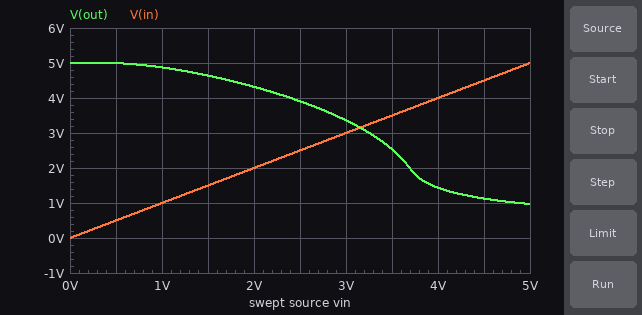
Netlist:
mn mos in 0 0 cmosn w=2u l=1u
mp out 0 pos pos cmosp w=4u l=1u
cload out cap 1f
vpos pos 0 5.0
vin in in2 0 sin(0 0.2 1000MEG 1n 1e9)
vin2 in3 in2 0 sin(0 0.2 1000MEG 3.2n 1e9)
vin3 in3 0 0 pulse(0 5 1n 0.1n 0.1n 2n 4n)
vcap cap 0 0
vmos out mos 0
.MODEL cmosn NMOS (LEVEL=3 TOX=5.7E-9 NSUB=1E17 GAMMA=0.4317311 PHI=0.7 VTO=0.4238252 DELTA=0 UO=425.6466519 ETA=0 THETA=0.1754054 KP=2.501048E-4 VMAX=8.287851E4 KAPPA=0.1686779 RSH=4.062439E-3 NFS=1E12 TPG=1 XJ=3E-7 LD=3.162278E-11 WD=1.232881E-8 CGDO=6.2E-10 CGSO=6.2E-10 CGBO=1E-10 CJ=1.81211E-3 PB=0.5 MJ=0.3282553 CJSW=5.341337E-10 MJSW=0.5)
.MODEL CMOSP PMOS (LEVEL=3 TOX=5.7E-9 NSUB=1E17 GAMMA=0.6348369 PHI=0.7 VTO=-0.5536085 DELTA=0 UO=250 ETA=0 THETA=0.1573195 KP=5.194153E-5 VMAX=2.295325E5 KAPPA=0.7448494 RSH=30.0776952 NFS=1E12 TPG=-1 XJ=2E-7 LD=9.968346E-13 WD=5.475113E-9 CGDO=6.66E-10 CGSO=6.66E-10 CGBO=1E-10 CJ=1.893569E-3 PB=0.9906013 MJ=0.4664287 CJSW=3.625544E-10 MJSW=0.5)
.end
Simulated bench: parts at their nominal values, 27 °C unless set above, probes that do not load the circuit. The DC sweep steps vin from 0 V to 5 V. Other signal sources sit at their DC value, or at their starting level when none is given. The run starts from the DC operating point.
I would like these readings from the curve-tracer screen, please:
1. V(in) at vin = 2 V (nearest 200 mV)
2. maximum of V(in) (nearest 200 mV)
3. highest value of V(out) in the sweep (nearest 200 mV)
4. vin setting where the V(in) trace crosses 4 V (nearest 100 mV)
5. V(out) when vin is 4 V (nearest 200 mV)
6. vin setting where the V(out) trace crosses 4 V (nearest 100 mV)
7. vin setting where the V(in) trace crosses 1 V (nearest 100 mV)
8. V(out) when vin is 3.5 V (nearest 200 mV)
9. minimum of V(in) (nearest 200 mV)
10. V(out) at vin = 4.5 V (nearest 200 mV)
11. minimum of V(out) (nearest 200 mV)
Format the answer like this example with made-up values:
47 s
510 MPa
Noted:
2.0 V
5.0 V
5.0 V
4.0 V
1.4 V
2.4 V
1.0 V
2.6 V
0 V
1.2 V
1.0 V
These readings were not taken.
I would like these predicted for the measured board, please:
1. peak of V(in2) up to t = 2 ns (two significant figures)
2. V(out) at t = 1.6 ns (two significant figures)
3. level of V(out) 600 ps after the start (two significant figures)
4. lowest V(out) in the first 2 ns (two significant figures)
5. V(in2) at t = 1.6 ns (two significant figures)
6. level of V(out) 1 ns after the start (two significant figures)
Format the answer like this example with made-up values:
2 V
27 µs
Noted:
5.0 V
980 mV
5.0 V
930 mV
5.0 V
5.0 V
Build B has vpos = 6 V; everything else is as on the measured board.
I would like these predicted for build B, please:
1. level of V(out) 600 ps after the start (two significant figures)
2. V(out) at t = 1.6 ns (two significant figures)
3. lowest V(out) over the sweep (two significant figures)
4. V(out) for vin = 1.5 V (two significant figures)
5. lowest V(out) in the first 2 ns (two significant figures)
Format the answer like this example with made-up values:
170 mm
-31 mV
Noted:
6.0 V
1.7 V
1.6 V
5.7 V
1.5 V
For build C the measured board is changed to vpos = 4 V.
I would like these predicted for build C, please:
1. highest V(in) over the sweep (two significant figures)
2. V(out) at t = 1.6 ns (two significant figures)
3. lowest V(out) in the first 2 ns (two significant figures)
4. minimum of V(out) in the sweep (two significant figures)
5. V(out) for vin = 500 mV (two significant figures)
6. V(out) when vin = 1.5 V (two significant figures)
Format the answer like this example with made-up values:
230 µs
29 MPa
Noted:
5.0 V
580 mV
560 mV
570 mV
4.0 V
3.6 V
